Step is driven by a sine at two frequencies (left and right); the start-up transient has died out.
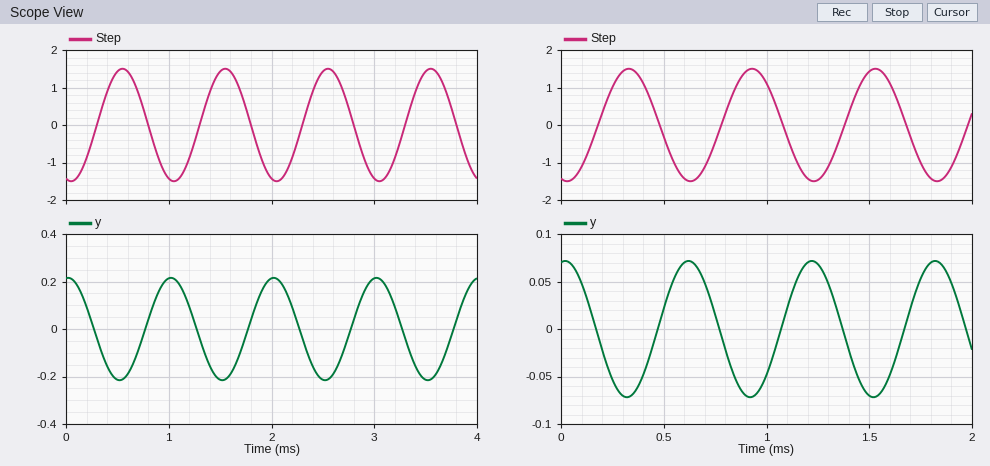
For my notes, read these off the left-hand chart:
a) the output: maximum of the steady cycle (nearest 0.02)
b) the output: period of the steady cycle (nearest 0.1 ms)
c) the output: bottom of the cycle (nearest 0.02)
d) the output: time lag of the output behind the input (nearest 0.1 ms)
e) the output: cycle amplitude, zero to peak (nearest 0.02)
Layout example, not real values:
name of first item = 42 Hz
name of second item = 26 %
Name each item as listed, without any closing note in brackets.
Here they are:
the output: maximum of the steady cycle = 0.22
the output: period of the steady cycle = 1.0 ms
the output: bottom of the cycle = -0.22
the output: time lag of the output behind the input = 0.5 ms
the output: cycle amplitude, zero to peak = 0.22
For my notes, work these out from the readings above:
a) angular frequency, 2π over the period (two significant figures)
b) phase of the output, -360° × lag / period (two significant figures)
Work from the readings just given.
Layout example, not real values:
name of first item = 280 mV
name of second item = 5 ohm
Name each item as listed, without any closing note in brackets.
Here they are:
angular frequency, 2π over the period = 6.3 rad/ms
phase of the output, -360° × lag / period = -180°
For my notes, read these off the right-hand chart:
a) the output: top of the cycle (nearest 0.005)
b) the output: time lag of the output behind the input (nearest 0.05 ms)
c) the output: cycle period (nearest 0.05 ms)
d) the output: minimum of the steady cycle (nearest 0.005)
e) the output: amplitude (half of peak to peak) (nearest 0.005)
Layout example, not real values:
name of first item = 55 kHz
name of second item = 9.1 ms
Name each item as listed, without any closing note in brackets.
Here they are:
the output: top of the cycle = 0.070
the output: time lag of the output behind the input = 0.30 ms
the output: cycle period = 0.60 ms
the output: minimum of the steady cycle = -0.070
the output: amplitude (half of peak to peak) = 0.070
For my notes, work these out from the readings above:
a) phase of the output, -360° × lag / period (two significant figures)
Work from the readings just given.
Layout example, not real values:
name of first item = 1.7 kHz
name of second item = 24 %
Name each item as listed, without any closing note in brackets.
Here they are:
phase of the output, -360° × lag / period = -180°
